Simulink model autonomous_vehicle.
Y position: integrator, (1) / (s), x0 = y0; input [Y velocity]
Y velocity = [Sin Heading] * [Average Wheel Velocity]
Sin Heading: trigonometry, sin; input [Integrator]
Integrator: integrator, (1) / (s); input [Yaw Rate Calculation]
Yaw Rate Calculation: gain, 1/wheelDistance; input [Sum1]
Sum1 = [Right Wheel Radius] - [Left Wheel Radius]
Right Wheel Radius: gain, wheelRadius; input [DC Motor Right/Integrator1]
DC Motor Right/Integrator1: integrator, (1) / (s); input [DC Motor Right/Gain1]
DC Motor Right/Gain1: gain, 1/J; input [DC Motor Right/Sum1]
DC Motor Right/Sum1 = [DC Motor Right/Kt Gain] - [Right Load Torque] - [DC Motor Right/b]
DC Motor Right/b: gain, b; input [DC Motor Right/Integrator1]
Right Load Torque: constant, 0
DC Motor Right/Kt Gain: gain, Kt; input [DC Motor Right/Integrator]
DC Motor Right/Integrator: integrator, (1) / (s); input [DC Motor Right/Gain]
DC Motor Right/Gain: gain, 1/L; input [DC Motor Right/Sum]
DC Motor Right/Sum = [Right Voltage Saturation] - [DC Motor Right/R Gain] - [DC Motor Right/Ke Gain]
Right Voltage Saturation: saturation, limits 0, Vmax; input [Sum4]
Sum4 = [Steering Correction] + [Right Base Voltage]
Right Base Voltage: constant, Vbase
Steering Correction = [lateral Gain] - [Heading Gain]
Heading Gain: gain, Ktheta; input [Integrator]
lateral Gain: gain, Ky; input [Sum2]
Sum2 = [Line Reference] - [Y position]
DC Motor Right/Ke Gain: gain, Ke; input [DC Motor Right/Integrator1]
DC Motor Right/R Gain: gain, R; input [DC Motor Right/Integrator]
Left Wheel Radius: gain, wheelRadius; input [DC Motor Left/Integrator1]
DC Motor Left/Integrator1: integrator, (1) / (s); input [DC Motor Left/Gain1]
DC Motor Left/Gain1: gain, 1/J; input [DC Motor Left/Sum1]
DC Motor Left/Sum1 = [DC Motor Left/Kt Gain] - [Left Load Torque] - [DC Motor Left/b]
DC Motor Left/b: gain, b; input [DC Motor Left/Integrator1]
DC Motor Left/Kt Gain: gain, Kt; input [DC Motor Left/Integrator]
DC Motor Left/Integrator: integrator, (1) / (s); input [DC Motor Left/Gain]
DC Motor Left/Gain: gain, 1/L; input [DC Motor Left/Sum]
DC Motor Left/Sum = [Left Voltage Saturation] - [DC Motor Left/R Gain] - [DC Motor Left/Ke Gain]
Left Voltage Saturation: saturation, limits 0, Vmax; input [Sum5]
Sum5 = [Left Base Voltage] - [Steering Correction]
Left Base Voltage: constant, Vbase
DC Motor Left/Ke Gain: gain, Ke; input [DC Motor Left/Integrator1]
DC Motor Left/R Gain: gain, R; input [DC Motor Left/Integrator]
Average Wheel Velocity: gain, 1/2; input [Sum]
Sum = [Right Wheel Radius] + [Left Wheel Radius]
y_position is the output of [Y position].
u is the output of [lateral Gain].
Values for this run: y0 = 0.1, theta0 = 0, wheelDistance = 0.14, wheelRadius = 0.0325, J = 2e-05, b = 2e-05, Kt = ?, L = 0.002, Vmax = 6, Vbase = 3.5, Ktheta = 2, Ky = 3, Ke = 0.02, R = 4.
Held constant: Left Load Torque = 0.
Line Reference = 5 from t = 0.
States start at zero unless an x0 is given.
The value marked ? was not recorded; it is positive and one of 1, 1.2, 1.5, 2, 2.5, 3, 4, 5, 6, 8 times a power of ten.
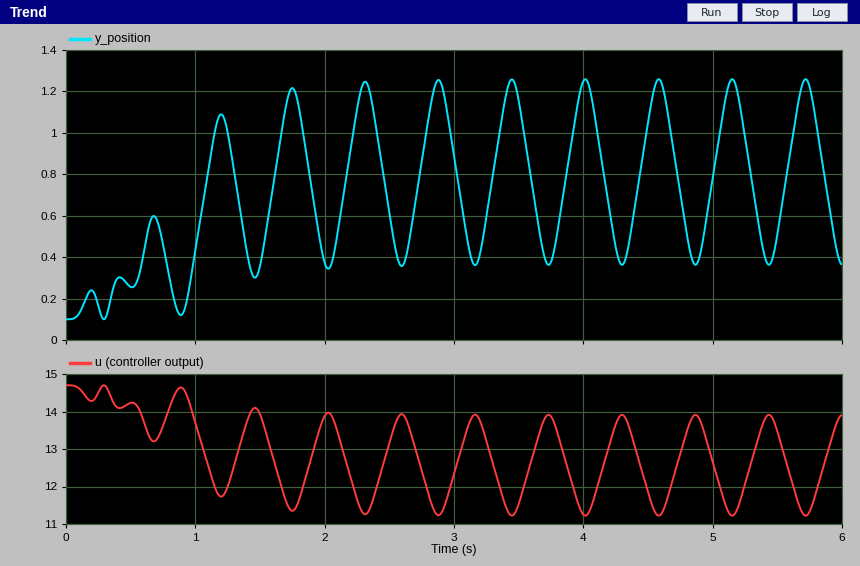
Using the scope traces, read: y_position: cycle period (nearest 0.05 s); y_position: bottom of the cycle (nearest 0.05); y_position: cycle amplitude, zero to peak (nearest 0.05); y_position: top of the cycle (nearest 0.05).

0.55 s
0.35
0.45
1.25
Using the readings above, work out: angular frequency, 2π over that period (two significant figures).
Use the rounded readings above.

11 rad/s
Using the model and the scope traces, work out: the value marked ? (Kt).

0.012
